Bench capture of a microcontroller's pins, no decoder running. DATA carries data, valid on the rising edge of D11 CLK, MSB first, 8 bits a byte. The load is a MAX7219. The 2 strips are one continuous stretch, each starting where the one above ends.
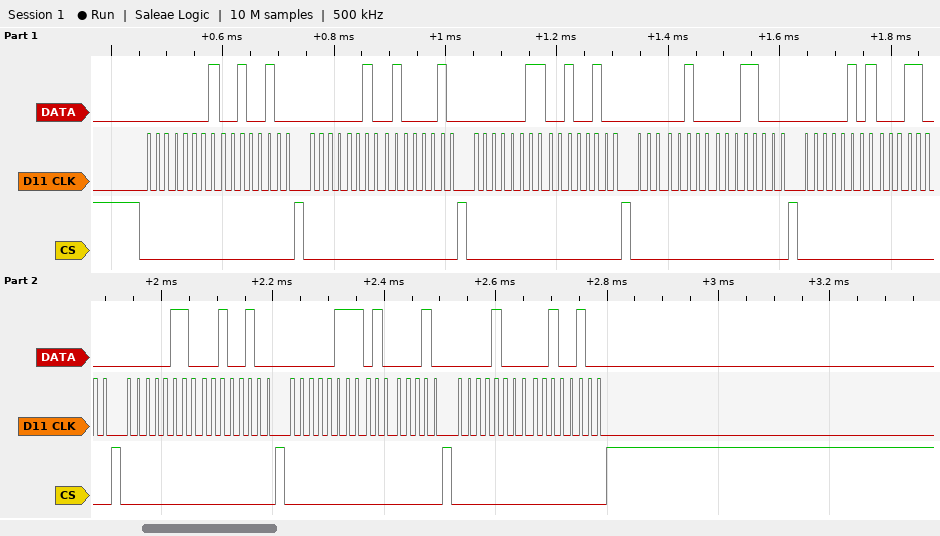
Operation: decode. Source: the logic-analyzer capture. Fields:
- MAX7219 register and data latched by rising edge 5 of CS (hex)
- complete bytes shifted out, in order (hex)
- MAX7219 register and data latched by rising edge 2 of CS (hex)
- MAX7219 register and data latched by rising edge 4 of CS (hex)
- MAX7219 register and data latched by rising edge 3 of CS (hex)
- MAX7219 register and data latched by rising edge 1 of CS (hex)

register 0x5, data 0x18
01 24 02 42 03 24 04 18 05 18 06 24 07 42 08 24
register 0x2, data 0x42
register 0x4, data 0x18
register 0x3, data 0x24
register 0x1, data 0x24
